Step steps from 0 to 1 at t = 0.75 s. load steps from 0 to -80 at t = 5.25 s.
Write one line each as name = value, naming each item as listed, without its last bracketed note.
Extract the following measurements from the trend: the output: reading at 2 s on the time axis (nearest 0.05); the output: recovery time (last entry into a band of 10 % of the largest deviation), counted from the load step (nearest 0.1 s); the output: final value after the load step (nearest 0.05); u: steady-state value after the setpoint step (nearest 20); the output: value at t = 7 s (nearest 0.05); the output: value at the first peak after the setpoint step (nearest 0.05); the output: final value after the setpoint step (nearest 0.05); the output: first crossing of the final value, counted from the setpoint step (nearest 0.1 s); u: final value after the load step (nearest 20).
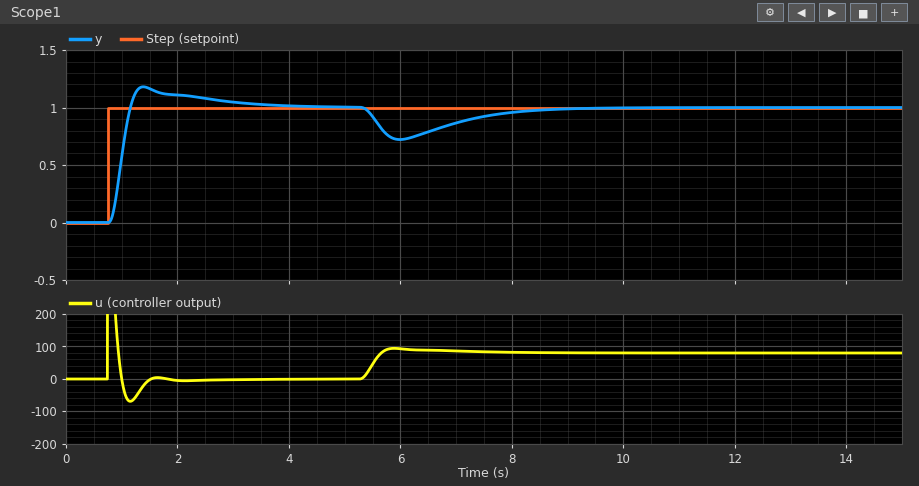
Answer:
the output: reading at 2 s on the time axis = 1.10
the output: recovery time (last entry into a band of 10 % of the largest deviation), counted from the load step = 3.1 s
the output: final value after the load step = 1.00
u: steady-state value after the setpoint step = 0
the output: value at t = 7 s = 0.85
the output: value at the first peak after the setpoint step = 1.20
the output: final value after the setpoint step = 1.00
the output: first crossing of the final value, counted from the setpoint step = 0.4 s
u: final value after the load step = 80
